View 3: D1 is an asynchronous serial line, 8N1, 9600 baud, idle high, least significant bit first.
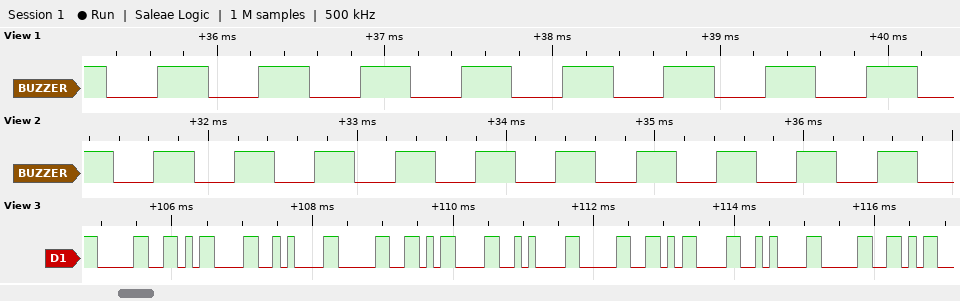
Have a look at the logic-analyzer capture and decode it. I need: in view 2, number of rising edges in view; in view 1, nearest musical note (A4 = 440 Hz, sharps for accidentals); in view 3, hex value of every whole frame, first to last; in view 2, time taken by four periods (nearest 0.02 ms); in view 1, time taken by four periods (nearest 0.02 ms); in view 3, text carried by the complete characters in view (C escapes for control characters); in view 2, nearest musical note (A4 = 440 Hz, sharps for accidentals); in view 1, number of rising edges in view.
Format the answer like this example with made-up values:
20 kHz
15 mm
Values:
10
G#6
30 0D 0A 30 0D 0A 30 0D 0A 30
2.16 ms
2.42 ms
"0\r\n0\r\n0\r\n0"
A#6
8
